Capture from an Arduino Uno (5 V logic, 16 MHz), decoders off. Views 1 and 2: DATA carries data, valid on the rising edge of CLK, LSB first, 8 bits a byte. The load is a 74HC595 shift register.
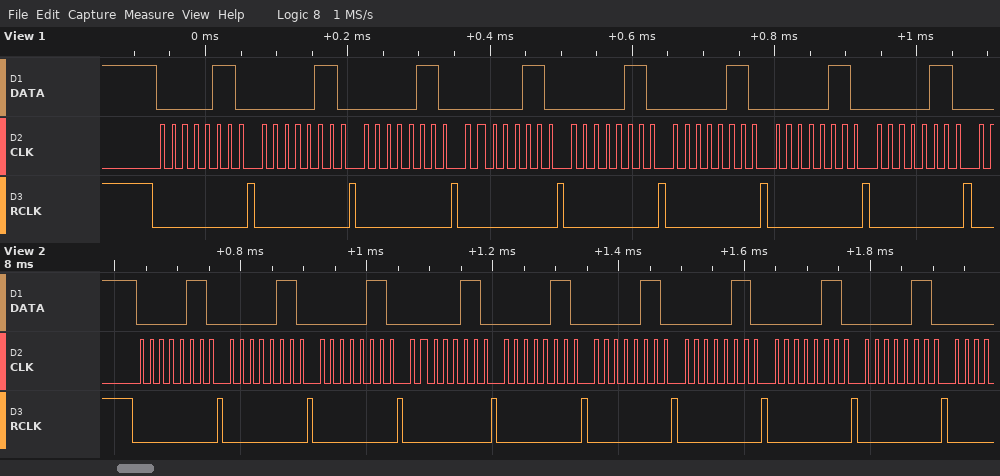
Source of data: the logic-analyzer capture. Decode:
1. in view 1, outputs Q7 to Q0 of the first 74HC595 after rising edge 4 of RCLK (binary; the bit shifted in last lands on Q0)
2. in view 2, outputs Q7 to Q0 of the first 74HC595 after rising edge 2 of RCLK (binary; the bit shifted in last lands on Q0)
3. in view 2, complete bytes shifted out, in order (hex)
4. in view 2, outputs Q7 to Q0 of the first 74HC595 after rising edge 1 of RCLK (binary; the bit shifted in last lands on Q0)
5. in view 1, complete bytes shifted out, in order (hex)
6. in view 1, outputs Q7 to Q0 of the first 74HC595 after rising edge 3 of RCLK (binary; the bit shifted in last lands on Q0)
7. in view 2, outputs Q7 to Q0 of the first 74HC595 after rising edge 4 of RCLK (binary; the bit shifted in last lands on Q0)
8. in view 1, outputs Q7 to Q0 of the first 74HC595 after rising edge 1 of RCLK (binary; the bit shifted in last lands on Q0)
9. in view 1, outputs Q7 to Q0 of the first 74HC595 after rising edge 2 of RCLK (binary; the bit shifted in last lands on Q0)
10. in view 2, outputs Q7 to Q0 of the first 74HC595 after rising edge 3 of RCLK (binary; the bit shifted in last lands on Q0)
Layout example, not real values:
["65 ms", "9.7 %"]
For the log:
["00000110", "00000110", "0x60 0x60 0x60 0x60 0x60 0x60 0x60 0x60 0x60", "00000110", "0x60 0x60 0x60 0x60 0x60 0x60 0x60 0x60", "00000110", "00000110", "00000110", "00000110", "00000110"]
